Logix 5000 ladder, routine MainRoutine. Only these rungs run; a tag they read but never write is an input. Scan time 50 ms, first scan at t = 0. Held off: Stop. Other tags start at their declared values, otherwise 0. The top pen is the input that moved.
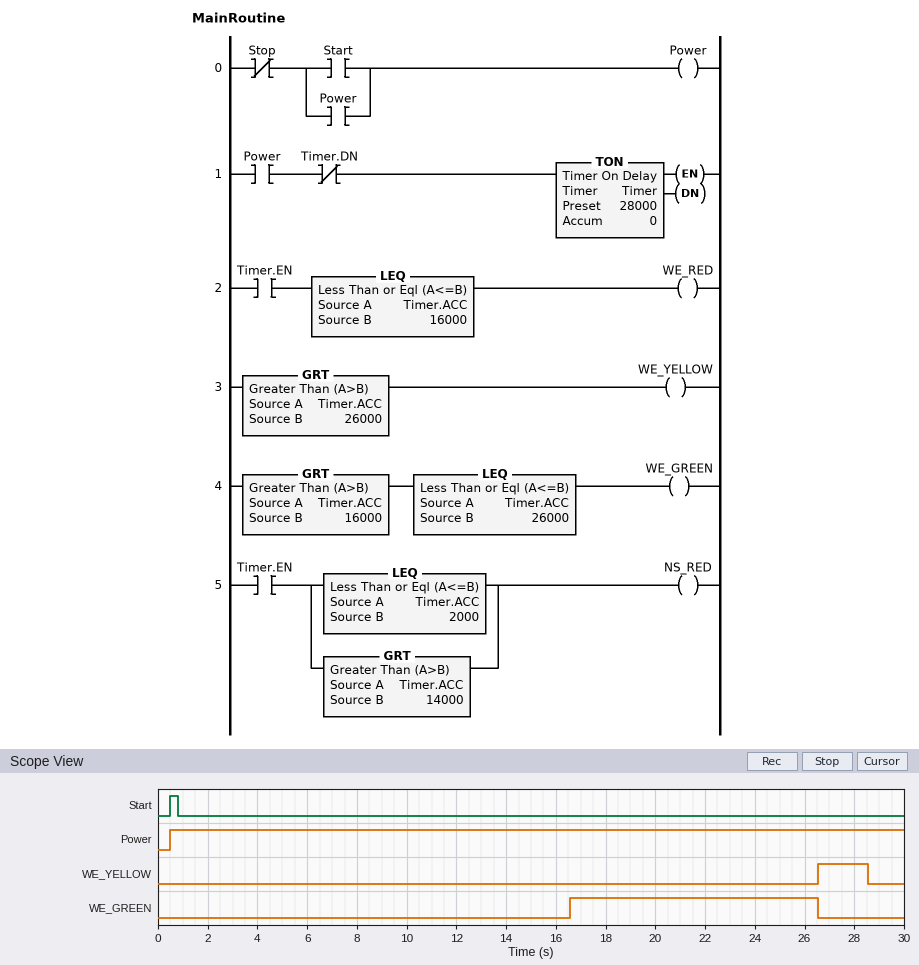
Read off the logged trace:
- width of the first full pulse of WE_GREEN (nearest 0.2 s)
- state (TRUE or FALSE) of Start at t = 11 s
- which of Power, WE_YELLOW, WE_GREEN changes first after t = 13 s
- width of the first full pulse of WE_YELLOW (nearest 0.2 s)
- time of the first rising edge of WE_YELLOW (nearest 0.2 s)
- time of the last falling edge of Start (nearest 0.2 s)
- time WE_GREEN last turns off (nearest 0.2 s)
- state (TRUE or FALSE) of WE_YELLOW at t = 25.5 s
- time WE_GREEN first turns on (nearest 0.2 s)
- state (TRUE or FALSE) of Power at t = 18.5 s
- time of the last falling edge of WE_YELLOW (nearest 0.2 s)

10.0 s
FALSE
WE_GREEN
2.0 s
26.6 s
0.8 s
26.6 s
FALSE
16.6 s
TRUE
28.6 s
